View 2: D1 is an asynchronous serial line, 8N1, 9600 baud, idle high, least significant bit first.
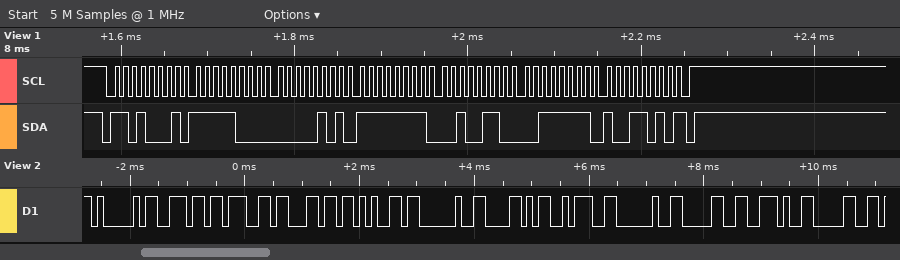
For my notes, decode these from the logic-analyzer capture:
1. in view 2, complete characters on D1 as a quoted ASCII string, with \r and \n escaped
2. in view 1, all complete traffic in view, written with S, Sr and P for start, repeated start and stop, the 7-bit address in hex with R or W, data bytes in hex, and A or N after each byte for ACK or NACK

"Angle X: 0.0"
S 68R A F8 A 05 A FF A 26 A 3F A 9A N P
